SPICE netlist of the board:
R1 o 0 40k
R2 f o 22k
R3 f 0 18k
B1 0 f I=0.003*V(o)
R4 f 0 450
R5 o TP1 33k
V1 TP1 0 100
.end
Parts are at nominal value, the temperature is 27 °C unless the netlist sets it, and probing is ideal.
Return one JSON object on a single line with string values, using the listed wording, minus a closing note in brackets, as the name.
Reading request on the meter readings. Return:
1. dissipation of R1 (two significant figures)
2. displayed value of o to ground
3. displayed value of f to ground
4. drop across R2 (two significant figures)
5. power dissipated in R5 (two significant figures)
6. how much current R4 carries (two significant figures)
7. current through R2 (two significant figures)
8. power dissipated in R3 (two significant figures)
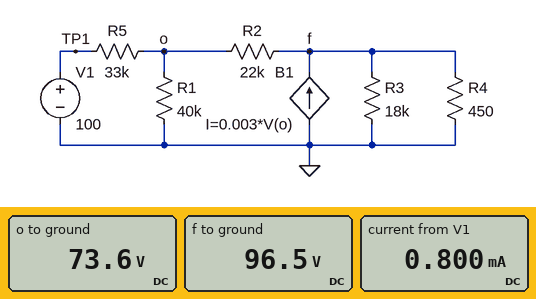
{"dissipation of R1": "140 mW", "displayed value of o to ground": "73.6 V", "displayed value of f to ground": "96.5 V", "drop across R2": "23 V", "power dissipated in R5": "21 mW", "how much current R4 carries": "210 mA", "current through R2": "1.0 mA", "power dissipated in R3": "520 mW"}
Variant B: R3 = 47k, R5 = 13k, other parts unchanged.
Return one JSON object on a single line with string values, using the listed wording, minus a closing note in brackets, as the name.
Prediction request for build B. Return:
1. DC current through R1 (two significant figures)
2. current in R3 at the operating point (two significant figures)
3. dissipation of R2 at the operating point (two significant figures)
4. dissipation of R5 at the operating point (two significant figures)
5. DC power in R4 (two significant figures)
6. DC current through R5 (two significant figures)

{"DC current through R1": "2.2 mA", "current in R3 at the operating point": "2.5 mA", "dissipation of R2 at the operating point": "39 mW", "dissipation of R5 at the operating point": "10 mW", "DC power in R4": "31 W", "DC current through R5": "880 µA"}
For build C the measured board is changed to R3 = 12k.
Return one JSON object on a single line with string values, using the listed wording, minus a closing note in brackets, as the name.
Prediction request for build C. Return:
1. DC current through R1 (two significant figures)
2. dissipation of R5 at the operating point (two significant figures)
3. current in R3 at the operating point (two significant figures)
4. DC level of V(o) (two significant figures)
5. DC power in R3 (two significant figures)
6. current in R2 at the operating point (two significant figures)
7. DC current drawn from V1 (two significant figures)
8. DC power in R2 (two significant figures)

{"DC current through R1": "1.8 mA", "dissipation of R5 at the operating point": "23 mW", "current in R3 at the operating point": "7.8 mA", "DC level of V(o)": "72 V", "DC power in R3": "730 mW", "current in R2 at the operating point": "970 µA", "DC current drawn from V1": "840 µA", "DC power in R2": "21 mW"}
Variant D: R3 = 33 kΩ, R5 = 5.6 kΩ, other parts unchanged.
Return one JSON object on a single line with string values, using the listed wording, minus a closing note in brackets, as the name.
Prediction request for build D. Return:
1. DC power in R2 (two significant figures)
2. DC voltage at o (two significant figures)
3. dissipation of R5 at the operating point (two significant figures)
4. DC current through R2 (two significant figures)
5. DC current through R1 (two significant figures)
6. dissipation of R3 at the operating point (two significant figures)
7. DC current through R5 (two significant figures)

{"DC power in R2": "43 mW", "DC voltage at o": "95 V", "dissipation of R5 at the operating point": "5.2 mW", "DC current through R2": "1.4 mA", "DC current through R1": "2.4 mA", "dissipation of R3 at the operating point": "480 mW", "DC current through R5": "970 µA"}
